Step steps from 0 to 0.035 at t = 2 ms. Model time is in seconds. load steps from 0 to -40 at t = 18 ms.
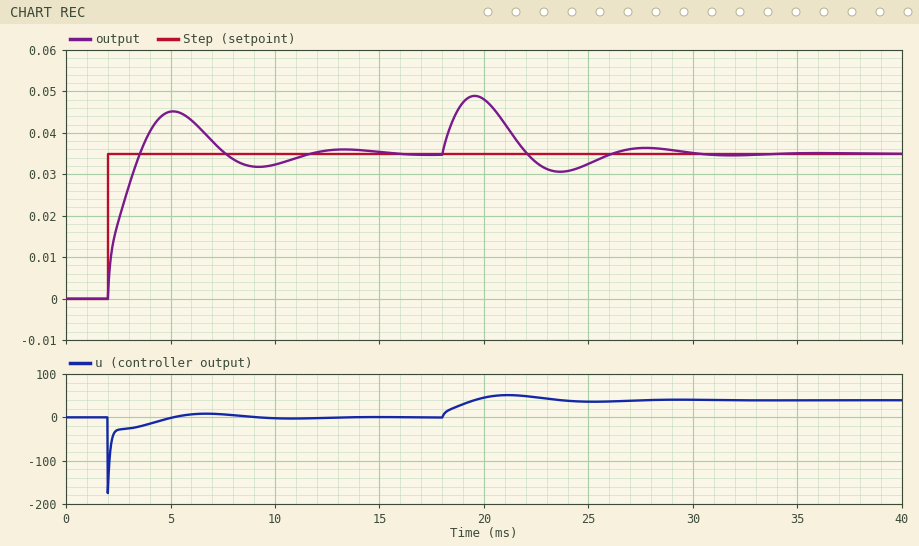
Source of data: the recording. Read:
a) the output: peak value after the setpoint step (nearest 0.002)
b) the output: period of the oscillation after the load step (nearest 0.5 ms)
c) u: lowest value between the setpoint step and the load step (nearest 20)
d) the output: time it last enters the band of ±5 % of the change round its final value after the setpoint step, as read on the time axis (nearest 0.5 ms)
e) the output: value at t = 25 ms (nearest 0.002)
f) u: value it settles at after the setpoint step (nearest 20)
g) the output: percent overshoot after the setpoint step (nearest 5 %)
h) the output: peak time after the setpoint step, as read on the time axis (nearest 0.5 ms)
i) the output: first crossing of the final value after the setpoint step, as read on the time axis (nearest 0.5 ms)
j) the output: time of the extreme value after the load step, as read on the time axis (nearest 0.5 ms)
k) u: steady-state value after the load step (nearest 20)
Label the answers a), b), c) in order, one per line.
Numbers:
a) 0.046
b) 8.0 ms
c) -180
d) 10.5 ms
e) 0.032
f) 0
g) 30 %
h) 5.0 ms
i) 3.5 ms
j) 19.5 ms
k) 40
